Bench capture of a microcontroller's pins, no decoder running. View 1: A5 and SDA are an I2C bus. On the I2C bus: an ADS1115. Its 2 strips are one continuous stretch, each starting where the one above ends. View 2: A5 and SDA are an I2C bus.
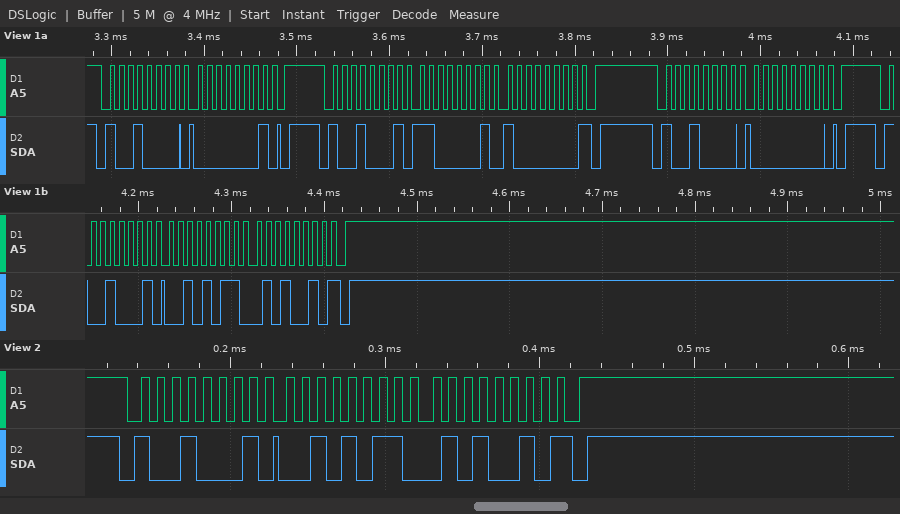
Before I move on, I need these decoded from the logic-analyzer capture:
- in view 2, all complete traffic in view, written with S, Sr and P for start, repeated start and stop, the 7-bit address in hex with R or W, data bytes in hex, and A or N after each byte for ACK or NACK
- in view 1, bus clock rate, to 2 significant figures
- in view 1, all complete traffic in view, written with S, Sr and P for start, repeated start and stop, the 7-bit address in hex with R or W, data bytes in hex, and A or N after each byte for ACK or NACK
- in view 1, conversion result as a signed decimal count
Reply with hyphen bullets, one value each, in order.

- S 48R A 2B A 52 N P
- 100 kHz
- S 48W A 01 A P S 48R A C1 A 80 N P S 48W A 00 A P S 48R A 2B A 52 N P
- 11090
